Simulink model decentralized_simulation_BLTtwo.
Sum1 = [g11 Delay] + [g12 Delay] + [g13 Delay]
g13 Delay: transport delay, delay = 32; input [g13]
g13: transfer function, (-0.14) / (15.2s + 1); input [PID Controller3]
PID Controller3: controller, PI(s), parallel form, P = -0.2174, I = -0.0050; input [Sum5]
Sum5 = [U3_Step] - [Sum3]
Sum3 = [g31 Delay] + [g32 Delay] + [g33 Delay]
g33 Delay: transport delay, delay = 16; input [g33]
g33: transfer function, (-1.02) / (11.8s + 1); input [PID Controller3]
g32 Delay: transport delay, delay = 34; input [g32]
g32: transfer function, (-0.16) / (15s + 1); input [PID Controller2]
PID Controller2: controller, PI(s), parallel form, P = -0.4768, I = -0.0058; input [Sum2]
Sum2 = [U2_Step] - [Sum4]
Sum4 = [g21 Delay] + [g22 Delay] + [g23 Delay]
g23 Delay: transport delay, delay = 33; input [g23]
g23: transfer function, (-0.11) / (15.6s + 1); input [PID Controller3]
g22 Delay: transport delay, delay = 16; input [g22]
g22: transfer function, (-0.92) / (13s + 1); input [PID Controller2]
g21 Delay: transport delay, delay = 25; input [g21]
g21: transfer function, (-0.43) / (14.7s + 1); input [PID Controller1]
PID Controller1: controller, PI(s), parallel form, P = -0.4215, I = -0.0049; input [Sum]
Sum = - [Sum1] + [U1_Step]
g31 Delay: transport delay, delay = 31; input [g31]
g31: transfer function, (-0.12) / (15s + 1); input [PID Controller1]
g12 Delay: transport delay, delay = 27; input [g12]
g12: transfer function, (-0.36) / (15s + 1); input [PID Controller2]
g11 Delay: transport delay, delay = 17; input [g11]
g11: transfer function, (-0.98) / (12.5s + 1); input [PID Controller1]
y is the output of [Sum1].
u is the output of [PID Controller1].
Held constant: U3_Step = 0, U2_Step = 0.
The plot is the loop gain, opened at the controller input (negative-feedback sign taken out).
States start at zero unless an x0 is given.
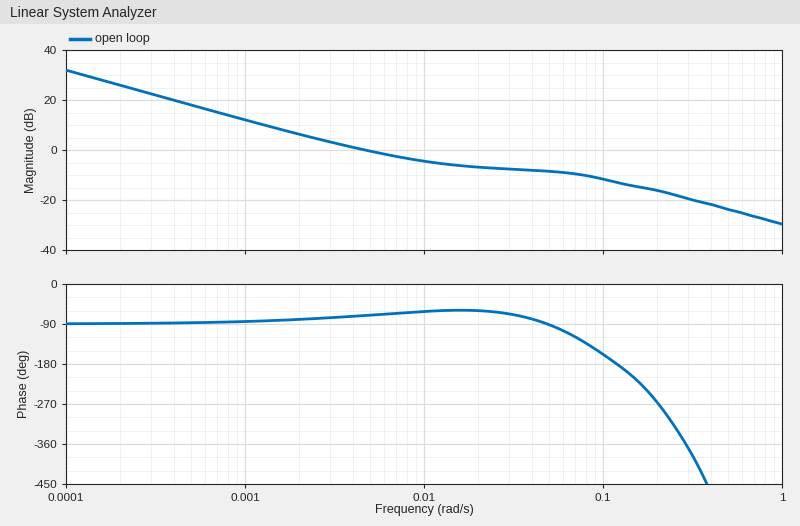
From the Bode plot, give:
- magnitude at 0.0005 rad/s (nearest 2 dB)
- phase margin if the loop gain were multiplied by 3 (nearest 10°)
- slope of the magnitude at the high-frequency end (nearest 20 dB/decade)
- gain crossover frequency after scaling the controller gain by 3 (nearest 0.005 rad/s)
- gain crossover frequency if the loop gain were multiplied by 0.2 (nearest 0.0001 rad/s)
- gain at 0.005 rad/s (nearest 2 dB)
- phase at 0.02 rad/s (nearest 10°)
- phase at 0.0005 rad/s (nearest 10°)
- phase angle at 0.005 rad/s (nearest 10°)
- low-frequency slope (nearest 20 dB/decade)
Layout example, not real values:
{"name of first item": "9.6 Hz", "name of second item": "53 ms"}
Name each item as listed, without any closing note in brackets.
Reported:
{"magnitude at 0.0005 rad/s": "18 dB", "phase margin if the loop gain were multiplied by 3": "60°", "slope of the magnitude at the high-frequency end": "-20 dB/decade", "gain crossover frequency after scaling the controller gain by 3": "0.070 rad/s", "gain crossover frequency if the loop gain were multiplied by 0.2": "0.0008 rad/s", "gain at 0.005 rad/s": "0 dB", "phase at 0.02 rad/s": "-60°", "phase at 0.0005 rad/s": "-90°", "phase angle at 0.005 rad/s": "-70°", "low-frequency slope": "-20 dB/decade"}
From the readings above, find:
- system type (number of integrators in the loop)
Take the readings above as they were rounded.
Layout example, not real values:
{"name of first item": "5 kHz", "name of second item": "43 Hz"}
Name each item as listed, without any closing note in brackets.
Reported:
{"system type": "1"}
